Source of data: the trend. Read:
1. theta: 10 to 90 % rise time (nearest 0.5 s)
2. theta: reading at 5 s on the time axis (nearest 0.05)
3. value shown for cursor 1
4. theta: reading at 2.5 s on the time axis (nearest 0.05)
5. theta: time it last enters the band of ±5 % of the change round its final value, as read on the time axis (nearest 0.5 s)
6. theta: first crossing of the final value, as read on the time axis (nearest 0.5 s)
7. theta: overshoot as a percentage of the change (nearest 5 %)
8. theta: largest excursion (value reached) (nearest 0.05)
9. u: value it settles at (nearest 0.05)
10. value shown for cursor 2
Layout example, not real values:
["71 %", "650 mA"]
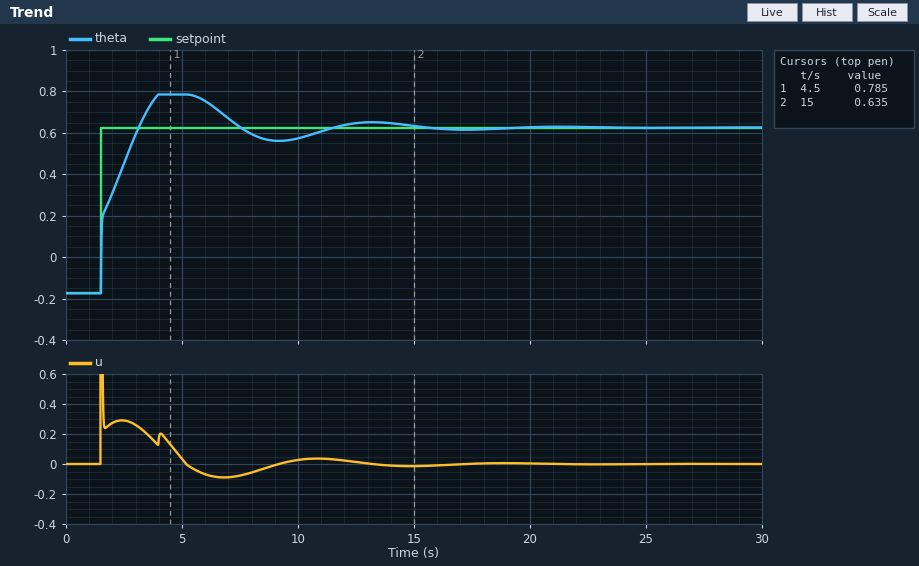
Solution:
["1.5 s", "0.80", "0.785", "0.45", "10.5 s", "3.0 s", "20 %", "0.80", "0.00", "0.635"]
